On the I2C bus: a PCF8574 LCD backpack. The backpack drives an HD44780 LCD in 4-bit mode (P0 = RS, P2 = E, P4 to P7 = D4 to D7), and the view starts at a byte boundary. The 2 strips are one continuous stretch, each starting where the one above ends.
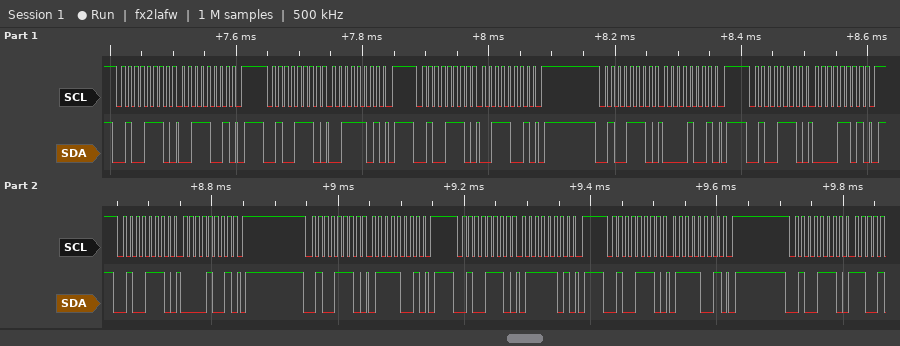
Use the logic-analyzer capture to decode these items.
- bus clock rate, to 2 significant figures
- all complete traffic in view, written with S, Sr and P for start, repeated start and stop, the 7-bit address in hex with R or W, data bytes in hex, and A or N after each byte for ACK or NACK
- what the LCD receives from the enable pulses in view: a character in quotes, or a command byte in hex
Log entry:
100 kHz
S 27W A 39 A P S 27W A 3D A P S 27W A 39 A P S 27W A 09 A P S 27W A 0D A P S 27W A 09 A P S 27W A 79 A P S 27W A 7D A P S 27W A 79 A P S 27W A
'0'
